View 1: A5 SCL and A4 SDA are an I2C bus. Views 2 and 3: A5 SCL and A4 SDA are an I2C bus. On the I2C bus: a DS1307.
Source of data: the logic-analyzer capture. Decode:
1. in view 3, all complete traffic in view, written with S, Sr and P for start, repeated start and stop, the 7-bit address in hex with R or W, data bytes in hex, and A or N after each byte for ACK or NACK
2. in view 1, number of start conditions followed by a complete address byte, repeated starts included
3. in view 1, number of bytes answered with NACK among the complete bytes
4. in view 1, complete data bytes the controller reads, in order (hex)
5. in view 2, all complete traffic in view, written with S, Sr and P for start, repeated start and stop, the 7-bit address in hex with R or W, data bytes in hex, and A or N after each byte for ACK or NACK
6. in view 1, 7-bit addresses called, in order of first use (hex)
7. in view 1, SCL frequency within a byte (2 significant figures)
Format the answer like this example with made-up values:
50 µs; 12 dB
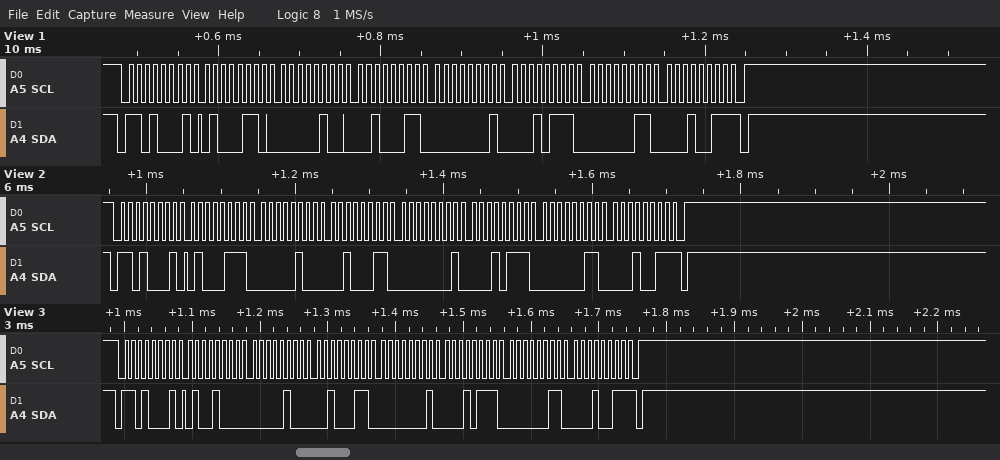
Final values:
S 68R A 48 A 04 A 23 A 01 A 17 A 03 A 13 N P; 1; 1; 46 04 23 01 17 03 13; S 68R A 47 A 04 A 23 A 01 A 17 A 03 A 13 N P; 0x68; 100 kHz
